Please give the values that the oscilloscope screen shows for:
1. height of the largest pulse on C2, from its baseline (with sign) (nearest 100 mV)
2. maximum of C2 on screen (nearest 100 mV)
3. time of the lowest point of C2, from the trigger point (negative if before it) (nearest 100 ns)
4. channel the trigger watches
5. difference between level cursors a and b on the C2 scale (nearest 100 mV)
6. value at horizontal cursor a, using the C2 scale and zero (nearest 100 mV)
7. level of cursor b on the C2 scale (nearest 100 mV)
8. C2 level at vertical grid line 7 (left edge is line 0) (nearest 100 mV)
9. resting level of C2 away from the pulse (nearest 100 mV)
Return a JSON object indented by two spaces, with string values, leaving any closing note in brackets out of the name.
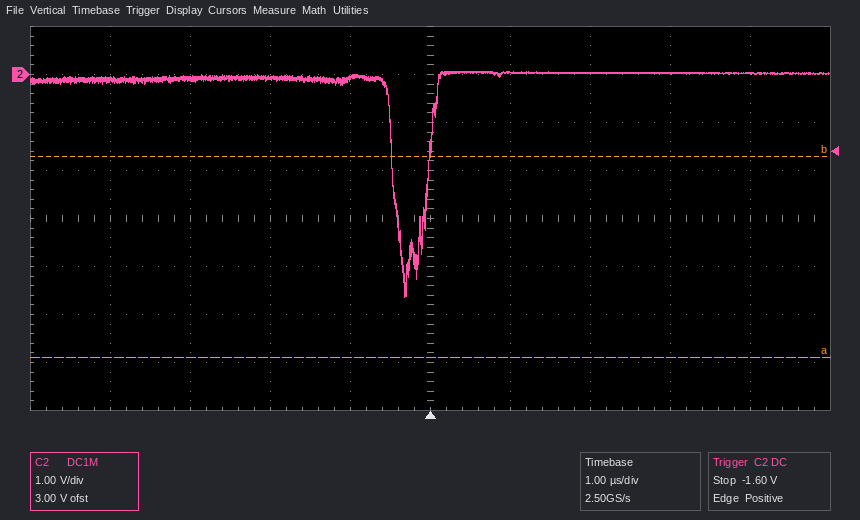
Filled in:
{
  "height of the largest pulse on C2, from its baseline (with sign)": "-4.7 V",
  "maximum of C2 on screen": "100 mV",
  "time of the lowest point of C2, from the trigger point (negative if before it)": "-300 ns",
  "channel the trigger watches": "C2",
  "difference between level cursors a and b on the C2 scale": "4.2 V",
  "value at horizontal cursor a, using the C2 scale and zero": "-5.9 V",
  "level of cursor b on the C2 scale": "-1.7 V",
  "C2 level at vertical grid line 7 (left edge is line 0)": "0.0 V",
  "resting level of C2 away from the pulse": "0.0 V"
}
